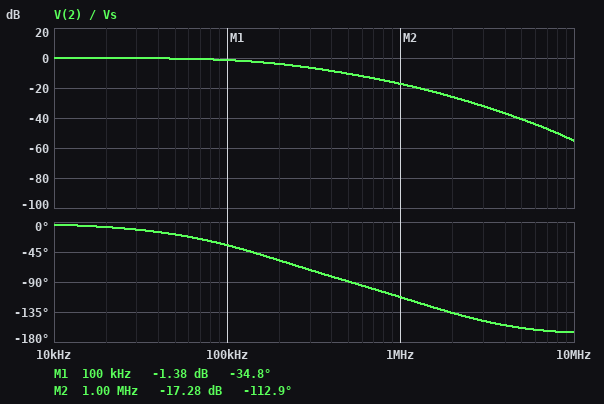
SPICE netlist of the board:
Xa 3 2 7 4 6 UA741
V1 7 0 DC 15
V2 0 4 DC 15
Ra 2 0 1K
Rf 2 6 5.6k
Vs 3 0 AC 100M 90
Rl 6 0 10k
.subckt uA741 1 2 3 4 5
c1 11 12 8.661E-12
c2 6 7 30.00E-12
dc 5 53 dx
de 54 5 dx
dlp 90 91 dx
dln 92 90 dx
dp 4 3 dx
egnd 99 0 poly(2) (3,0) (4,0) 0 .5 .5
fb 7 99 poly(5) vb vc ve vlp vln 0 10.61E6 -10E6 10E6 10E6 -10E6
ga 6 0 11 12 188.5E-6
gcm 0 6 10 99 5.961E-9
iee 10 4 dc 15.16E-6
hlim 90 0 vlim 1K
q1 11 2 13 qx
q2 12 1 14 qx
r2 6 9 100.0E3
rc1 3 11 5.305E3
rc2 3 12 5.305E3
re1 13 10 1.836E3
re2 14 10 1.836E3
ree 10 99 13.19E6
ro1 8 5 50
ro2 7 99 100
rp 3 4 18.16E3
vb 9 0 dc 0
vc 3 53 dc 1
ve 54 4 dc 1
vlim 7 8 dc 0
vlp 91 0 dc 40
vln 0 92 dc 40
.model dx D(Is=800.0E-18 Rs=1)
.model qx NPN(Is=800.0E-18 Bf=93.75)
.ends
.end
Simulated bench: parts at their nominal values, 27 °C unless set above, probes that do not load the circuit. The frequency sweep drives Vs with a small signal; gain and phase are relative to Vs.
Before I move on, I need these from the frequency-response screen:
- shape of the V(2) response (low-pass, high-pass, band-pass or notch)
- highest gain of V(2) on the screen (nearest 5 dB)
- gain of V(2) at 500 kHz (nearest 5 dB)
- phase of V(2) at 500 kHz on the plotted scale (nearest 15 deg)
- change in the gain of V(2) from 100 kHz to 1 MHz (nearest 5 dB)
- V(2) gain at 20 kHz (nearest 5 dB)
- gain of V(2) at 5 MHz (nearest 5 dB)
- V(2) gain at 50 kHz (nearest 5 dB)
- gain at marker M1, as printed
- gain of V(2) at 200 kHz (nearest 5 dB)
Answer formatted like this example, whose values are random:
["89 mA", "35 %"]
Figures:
["low-pass", "0 dB", "-10 dB", "-90 deg", "-15 dB", "0 dB", "-40 dB", "0 dB", "-1.38 dB", "-5 dB"]
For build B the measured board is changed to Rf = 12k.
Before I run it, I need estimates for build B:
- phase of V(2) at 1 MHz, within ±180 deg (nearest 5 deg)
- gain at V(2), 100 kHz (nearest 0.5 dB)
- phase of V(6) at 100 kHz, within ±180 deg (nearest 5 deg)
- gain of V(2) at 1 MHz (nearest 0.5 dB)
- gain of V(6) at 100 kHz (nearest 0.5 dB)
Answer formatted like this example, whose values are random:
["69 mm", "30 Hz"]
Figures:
["-115 deg", "-4.0 dB", "-55 deg", "-23.5 dB", "18.0 dB"]
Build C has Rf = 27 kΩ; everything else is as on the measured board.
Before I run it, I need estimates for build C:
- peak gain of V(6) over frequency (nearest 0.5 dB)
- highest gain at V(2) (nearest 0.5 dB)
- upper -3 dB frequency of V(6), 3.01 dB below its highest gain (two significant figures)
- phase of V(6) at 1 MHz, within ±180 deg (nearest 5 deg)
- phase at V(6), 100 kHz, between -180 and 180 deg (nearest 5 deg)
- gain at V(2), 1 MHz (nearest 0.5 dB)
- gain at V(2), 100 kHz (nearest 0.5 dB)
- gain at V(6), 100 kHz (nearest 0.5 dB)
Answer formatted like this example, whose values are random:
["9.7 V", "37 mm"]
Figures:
["29.0 dB", "0 dB", "36 kHz", "-120 deg", "-75 deg", "-30.5 dB", "-9.5 dB", "19.5 dB"]
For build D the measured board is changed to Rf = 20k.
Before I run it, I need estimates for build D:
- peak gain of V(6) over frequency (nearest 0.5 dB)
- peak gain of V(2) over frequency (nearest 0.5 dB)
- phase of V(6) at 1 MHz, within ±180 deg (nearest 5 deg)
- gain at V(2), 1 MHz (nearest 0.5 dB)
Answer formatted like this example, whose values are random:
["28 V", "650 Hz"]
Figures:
["26.5 dB", "0 dB", "-120 deg", "-27.5 dB"]
